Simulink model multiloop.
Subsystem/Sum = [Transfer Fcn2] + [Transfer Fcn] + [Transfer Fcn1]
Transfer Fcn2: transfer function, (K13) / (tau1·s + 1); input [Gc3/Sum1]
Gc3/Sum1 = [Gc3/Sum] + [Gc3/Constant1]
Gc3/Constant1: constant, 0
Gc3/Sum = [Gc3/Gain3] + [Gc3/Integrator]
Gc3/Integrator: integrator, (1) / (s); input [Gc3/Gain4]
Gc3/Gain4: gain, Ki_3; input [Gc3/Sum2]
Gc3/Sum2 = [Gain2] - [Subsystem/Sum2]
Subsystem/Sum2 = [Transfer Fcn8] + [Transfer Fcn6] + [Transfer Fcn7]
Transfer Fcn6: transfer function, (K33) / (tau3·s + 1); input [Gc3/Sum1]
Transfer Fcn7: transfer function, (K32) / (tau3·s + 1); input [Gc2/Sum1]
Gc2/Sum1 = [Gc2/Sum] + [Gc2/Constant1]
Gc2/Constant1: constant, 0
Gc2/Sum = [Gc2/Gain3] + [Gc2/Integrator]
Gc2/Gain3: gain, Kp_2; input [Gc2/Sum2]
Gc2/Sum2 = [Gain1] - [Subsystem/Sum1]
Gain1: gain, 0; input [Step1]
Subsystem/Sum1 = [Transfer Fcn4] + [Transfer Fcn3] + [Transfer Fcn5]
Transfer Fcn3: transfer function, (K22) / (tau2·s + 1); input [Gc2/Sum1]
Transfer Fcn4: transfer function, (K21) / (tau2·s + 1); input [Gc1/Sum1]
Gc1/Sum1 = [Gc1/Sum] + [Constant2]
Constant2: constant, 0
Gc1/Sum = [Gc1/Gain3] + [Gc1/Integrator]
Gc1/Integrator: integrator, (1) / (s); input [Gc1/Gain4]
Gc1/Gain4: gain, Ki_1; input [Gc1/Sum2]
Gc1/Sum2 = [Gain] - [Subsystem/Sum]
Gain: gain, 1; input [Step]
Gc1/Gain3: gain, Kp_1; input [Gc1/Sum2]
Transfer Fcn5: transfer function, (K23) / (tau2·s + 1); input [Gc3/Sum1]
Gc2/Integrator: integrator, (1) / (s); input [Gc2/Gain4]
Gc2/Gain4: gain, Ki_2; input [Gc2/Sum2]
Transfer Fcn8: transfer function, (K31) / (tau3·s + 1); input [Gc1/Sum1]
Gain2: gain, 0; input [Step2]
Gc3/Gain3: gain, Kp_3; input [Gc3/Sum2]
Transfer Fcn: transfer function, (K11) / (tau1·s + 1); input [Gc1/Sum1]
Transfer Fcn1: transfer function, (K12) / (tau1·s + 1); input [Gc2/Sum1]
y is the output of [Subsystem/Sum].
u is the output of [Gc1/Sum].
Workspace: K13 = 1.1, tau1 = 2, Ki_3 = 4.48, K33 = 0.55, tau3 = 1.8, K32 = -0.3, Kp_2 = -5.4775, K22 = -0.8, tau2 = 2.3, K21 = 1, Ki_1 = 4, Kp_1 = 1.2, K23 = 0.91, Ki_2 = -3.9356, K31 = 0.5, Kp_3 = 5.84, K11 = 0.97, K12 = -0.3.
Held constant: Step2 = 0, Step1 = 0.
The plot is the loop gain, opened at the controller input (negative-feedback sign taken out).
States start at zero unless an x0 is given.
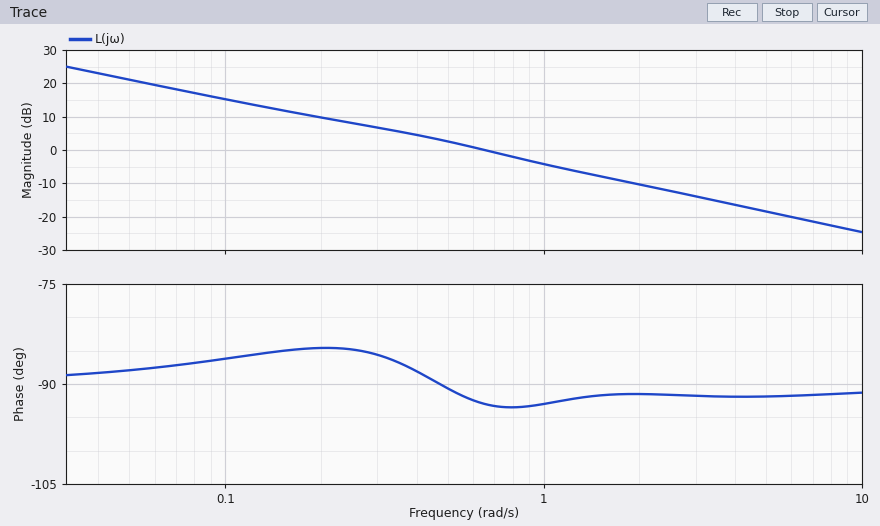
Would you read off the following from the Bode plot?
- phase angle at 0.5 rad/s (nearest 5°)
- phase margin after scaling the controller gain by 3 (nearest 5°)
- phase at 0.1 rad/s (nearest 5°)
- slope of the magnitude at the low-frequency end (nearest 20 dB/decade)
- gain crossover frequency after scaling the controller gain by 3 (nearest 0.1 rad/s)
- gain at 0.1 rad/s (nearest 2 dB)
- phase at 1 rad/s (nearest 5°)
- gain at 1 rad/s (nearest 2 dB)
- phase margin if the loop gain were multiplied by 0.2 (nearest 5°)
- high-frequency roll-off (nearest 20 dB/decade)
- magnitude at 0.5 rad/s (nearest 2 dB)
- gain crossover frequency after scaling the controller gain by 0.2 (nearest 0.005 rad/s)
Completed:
-90°
90°
-85°
-20 dB/decade
1.8 rad/s
16 dB
-95°
-4 dB
95°
-20 dB/decade
2 dB
0.115 rad/s
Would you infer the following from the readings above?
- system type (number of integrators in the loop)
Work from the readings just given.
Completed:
1
